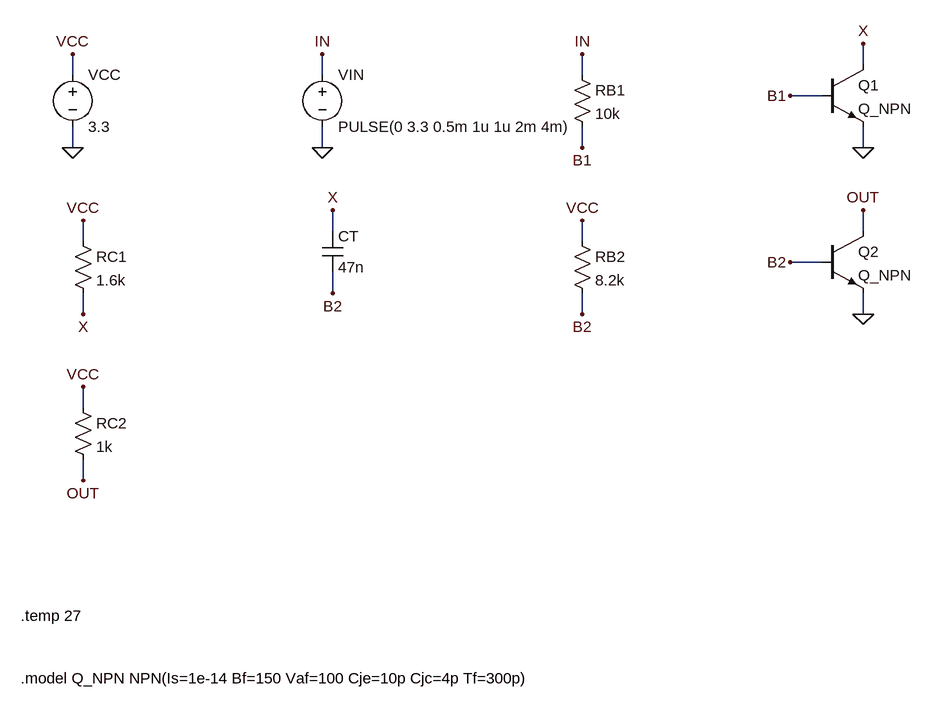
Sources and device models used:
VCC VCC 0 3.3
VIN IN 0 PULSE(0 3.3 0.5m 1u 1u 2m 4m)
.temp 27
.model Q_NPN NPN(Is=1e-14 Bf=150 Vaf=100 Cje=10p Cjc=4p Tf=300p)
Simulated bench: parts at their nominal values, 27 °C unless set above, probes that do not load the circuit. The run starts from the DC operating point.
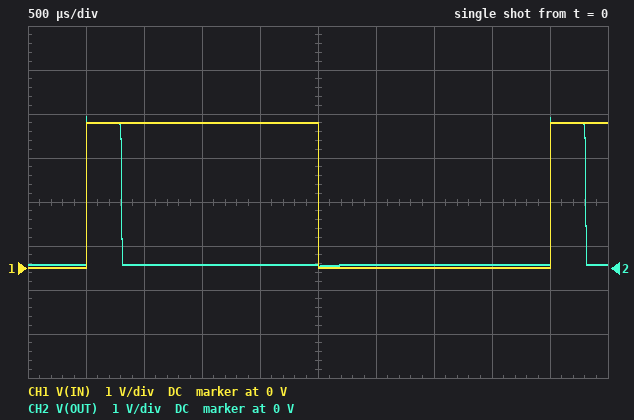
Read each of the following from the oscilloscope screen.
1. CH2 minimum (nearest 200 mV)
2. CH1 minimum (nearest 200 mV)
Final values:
0 V
0 V
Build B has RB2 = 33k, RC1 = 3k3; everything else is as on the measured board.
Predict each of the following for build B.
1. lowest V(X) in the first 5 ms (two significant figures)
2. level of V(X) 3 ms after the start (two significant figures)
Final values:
46 mV
3.2 V
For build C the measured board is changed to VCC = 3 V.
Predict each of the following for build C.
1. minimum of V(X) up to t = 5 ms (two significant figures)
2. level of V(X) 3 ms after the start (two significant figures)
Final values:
58 mV
3.0 V
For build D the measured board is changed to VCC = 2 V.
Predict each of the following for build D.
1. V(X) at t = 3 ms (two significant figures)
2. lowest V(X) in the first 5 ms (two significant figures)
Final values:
2.0 V
50 mV
